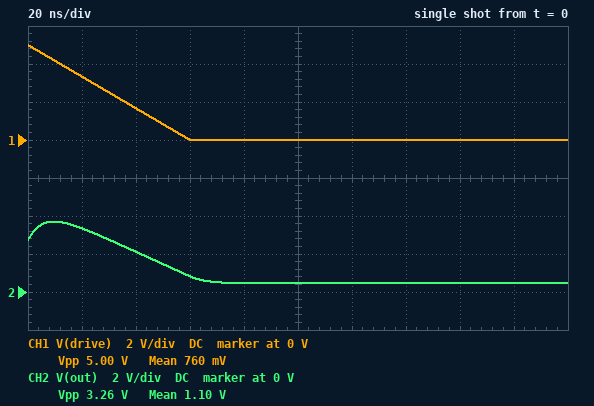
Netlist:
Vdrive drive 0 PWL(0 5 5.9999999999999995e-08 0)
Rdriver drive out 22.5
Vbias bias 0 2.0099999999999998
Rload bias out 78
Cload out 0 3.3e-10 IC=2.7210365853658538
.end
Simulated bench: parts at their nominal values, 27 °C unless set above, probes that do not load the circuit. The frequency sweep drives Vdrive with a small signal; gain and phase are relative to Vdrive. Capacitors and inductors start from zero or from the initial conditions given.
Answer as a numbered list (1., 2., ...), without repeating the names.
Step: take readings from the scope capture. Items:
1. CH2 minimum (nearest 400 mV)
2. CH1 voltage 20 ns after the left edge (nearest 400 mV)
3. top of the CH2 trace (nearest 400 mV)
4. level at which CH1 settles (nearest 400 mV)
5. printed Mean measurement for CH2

1. 400 mV
2. 3.2 V
3. 3.6 V
4. 0 V
5. 1.10 V
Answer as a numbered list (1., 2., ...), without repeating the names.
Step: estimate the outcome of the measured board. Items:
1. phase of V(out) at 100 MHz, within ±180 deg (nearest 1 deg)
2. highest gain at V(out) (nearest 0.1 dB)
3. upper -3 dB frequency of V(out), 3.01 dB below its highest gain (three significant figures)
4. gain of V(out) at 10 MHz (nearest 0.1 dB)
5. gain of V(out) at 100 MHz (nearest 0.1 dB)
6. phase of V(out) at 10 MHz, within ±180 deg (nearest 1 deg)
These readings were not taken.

1. -75 deg
2. -2.2 dB
3. 27.6 MHz
4. -2.7 dB
5. -13.7 dB
6. -20 deg
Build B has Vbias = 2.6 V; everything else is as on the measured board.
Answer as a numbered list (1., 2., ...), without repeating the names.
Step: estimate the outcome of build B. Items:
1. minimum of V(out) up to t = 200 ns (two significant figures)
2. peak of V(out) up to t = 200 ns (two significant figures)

1. 580 mV
2. 3.8 V
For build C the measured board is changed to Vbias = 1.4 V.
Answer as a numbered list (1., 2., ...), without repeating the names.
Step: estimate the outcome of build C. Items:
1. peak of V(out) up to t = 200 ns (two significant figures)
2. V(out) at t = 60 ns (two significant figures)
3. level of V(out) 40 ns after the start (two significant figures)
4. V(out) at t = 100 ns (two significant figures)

1. 3.6 V
2. 690 mV
3. 2.0 V
4. 310 mV
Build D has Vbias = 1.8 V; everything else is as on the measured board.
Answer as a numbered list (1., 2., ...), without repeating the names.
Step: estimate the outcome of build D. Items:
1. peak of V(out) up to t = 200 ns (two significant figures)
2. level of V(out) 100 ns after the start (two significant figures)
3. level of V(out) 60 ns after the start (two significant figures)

1. 3.7 V
2. 400 mV
3. 780 mV
